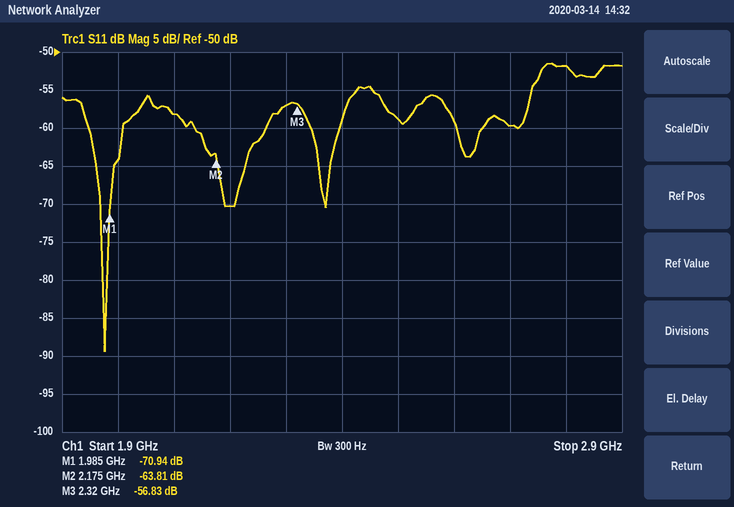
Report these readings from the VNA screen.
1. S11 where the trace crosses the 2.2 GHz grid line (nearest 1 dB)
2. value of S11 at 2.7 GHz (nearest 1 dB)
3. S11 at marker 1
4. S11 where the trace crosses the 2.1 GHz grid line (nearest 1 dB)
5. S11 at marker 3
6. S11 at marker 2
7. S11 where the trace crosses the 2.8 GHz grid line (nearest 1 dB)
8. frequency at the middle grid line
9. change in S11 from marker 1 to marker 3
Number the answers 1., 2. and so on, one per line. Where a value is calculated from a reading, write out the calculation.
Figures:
1. -70 dB
2. -60 dB
3. -70.94 dB
4. -58 dB
5. -56.83 dB
6. -63.81 dB
7. -52 dB
8. 2.4 GHz
9. -56.83 − (-70.94) = 14.11 dB
